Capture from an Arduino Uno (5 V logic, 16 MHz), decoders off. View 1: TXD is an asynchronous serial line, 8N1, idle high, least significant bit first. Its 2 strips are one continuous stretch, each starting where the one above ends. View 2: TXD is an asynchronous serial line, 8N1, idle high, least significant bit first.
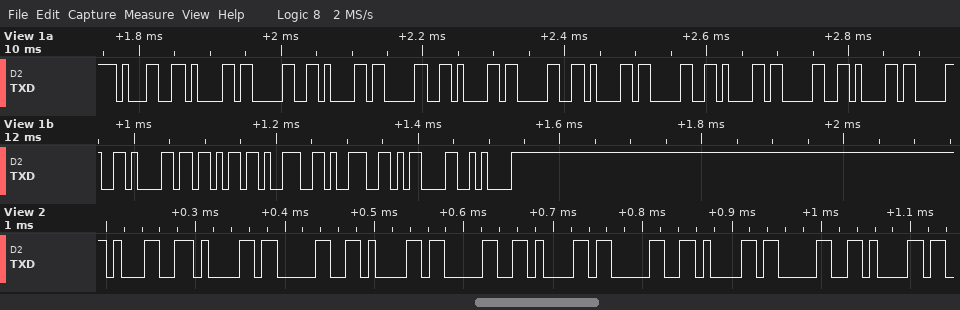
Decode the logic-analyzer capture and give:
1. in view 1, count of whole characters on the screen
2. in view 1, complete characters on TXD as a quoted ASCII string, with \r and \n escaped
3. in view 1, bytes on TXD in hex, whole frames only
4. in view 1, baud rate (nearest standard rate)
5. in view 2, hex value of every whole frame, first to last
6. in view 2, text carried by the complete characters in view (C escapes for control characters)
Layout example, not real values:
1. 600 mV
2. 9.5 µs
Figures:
1. 19
2. "1a0a0a0a0a0a0ak99\r\n"
3. 31 61 30 61 30 61 30 61 30 61 30 61 30 61 6B 39 39 0D 0A
4. 115200 baud
5. 31 61 30 61 30 61 30 61 30 61
6. "1a0a0a0a0a"
